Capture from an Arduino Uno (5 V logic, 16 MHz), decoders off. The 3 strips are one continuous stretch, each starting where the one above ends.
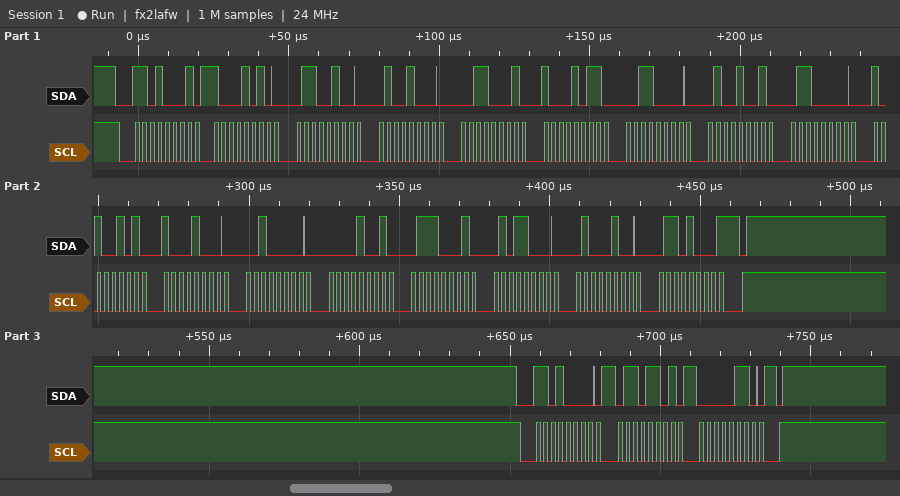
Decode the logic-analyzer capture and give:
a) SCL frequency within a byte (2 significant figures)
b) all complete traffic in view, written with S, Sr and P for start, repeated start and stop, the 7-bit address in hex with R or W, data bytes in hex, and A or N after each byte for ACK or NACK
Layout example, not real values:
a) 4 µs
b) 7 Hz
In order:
a) 400 kHz
b) S 68R A 8A A 64 A 48 A 31 A 8B A 30 A 49 A 60 A A5 A 88 A 20 A 09 A 71 A 58 A 44 A 68 N P S 68W A 6D A 06 A P
